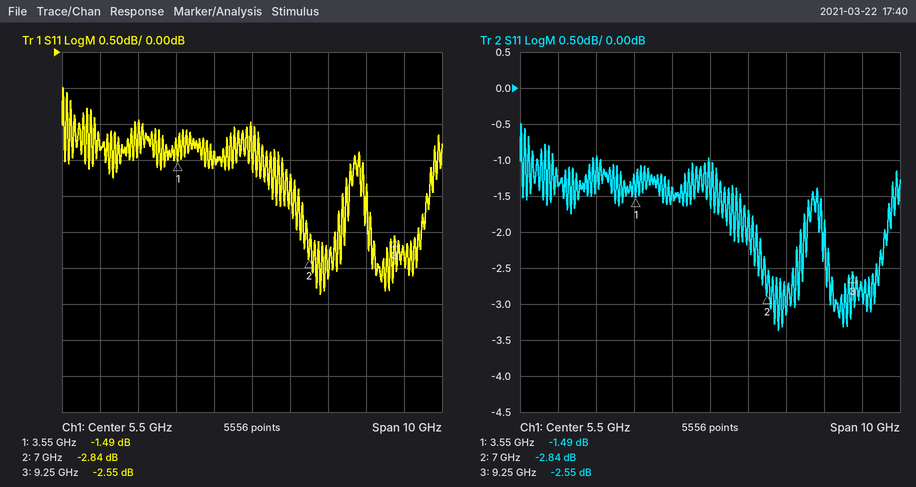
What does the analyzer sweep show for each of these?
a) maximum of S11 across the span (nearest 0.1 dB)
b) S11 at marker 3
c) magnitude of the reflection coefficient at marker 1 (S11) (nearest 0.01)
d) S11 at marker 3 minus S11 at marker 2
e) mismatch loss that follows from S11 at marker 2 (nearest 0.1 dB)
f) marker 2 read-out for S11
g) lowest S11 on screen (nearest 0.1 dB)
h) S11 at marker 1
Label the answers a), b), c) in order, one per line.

a) -0.5 dB
b) -2.55 dB
c) 0.84
d) 0.29 dB
e) 3.2 dB
f) -2.84 dB
g) -3.4 dB
h) -1.49 dB
